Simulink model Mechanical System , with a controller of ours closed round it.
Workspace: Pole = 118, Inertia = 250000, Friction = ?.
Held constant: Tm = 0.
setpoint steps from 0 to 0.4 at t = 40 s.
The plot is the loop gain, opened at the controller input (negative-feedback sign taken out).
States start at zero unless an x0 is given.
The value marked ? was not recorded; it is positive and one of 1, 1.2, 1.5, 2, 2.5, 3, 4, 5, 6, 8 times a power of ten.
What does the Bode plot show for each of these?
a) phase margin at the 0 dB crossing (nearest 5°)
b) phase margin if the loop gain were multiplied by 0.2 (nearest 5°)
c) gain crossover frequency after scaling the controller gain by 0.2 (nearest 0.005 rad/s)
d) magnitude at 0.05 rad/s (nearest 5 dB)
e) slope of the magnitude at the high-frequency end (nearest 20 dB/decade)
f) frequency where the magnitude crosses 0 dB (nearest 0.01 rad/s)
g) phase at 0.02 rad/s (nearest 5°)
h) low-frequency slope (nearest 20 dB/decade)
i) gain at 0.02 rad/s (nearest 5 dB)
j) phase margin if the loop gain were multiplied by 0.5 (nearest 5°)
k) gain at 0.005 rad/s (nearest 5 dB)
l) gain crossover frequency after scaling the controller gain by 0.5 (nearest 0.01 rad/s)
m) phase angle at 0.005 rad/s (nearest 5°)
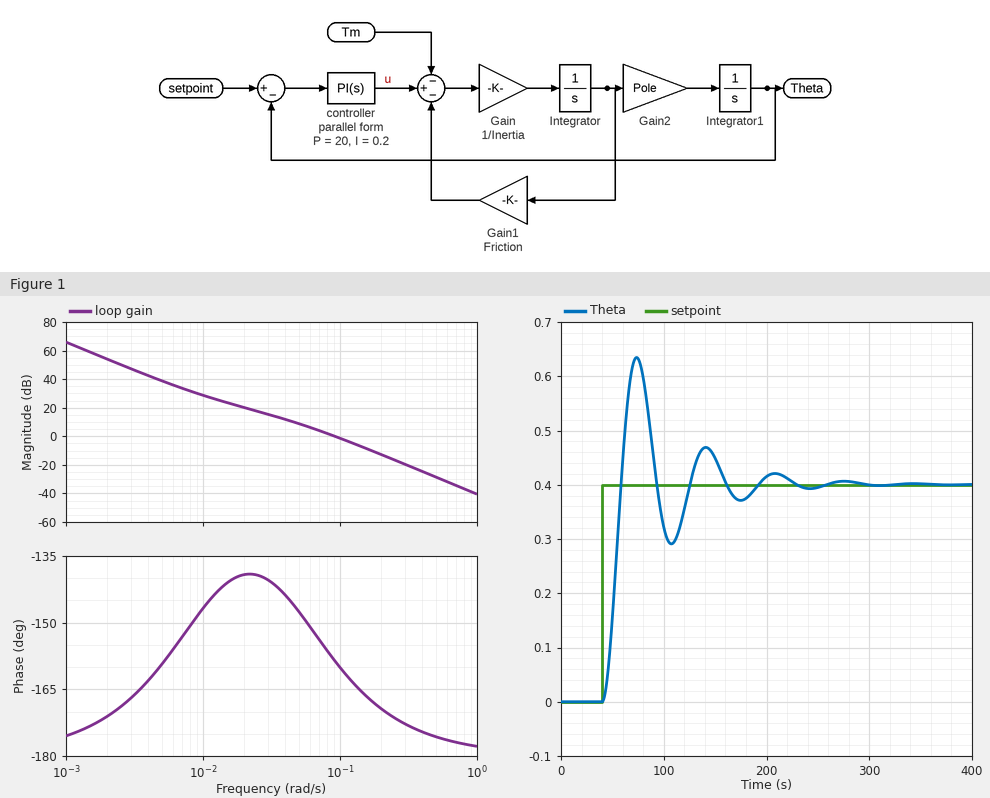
20°
40°
0.035 rad/s
10 dB
-40 dB/decade
0.09 rad/s
-140°
-40 dB/decade
20 dB
30°
40 dB
0.06 rad/s
-160°
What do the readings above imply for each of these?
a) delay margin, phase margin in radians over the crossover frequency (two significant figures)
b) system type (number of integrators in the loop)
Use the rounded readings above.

3.9 s
2
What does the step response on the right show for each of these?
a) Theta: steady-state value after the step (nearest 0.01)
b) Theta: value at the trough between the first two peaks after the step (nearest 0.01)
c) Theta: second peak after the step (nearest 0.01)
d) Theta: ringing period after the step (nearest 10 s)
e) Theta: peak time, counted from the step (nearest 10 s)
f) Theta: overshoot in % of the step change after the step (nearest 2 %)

0.40
0.29
0.47
70 s
30 s
58 %
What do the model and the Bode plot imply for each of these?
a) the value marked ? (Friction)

12000
